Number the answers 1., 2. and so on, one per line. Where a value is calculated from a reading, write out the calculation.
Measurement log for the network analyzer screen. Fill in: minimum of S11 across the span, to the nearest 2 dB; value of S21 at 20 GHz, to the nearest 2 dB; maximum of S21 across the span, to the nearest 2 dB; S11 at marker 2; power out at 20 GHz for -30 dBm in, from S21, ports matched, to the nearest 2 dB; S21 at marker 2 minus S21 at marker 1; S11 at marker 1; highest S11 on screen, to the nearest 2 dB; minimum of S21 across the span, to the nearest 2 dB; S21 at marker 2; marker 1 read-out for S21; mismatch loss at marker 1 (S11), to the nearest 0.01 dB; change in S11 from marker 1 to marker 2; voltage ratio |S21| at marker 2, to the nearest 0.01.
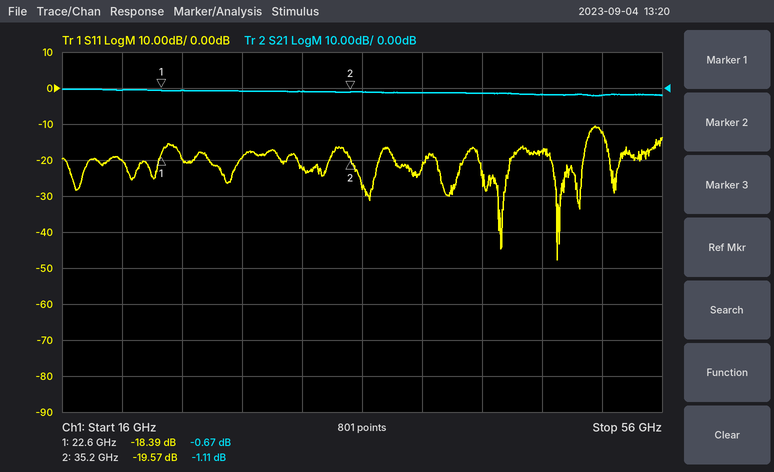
1. -48 dB
2. 0 dB
3. 0 dB
4. -19.57 dB
5. -30 dBm + (0 dB) = -30 dBm
6. -1.11 − (-0.67) = -0.44 dB
7. -18.39 dB
8. -10 dB
9. -2 dB
10. -1.11 dB
11. -0.67 dB
12. −10 log10(1 − 10^(-18.39/10)) ≈ 0.06 dB
13. -19.57 − (-18.39) = -1.18 dB
14. 10^(-1.11/20) ≈ 0.88
